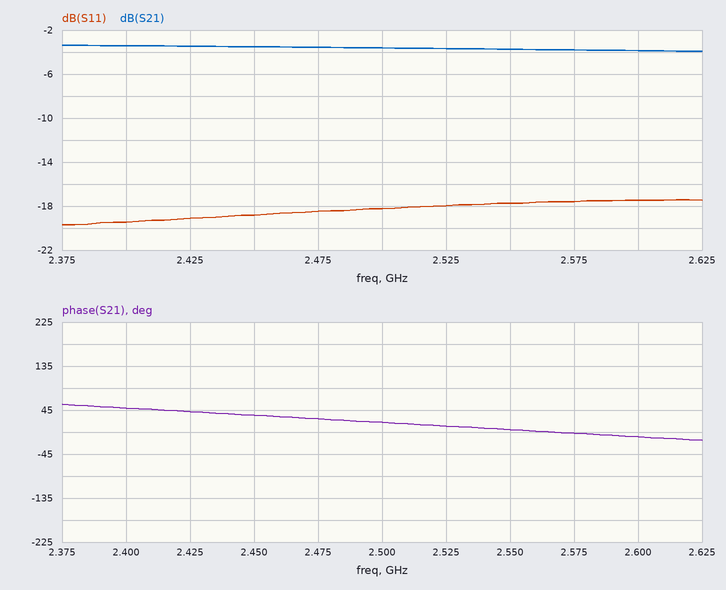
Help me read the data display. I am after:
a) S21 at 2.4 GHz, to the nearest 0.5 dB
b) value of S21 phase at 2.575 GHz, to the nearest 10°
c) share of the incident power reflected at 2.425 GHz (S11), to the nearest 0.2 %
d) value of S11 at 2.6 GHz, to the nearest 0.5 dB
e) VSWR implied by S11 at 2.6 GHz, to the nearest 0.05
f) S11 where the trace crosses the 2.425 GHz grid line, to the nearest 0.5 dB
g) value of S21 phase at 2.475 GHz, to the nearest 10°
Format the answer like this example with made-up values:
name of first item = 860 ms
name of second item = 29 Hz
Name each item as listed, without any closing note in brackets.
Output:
S21 at 2.4 GHz, to the nearest 0.5 dB = -3.5 dB
value of S21 phase at 2.575 GHz, to the nearest 10° = 0°
share of the incident power reflected at 2.425 GHz (S11), to the nearest 0.2 % = 1.2 %
value of S11 at 2.6 GHz, to the nearest 0.5 dB = -17.5 dB
VSWR implied by S11 at 2.6 GHz, to the nearest 0.05 = 1.30
S11 where the trace crosses the 2.425 GHz grid line, to the nearest 0.5 dB = -19.0 dB
value of S21 phase at 2.475 GHz, to the nearest 10° = 30°
